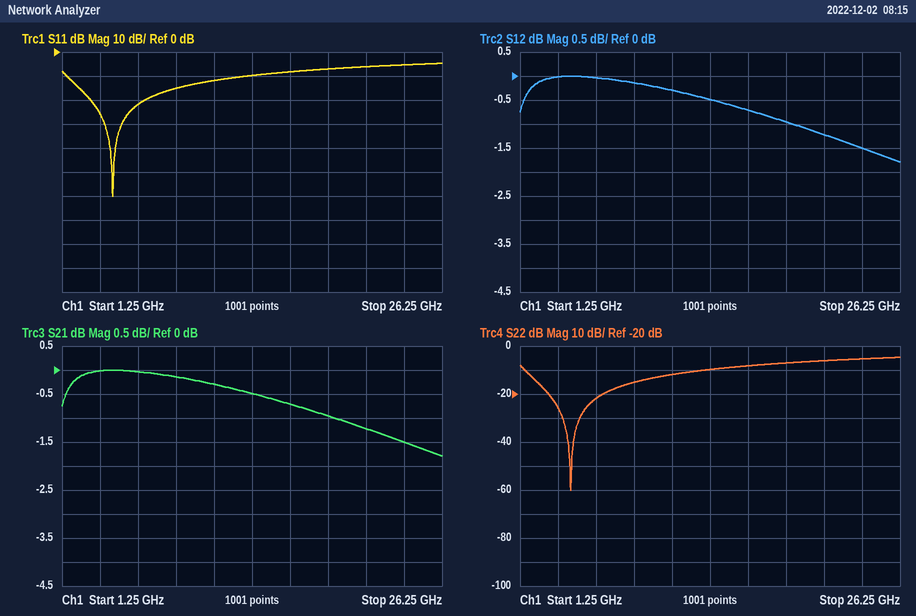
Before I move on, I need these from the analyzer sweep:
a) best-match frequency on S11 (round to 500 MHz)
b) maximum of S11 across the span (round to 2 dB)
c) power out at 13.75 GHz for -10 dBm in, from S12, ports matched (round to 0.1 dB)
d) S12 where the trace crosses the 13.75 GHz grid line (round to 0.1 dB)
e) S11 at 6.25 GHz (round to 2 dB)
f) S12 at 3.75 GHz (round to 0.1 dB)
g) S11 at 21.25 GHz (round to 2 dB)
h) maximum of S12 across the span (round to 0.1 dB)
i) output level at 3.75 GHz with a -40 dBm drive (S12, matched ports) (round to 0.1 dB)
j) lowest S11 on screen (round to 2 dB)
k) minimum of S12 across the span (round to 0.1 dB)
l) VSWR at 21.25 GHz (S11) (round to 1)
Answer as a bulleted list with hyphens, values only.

- 4.5 GHz
- -4 dB
- -10.5 dBm
- -0.5 dB
- -22 dB
- 0.0 dB
- -6 dB
- 0.0 dB
- -40.0 dBm
- -60 dB
- -1.8 dB
- 3
